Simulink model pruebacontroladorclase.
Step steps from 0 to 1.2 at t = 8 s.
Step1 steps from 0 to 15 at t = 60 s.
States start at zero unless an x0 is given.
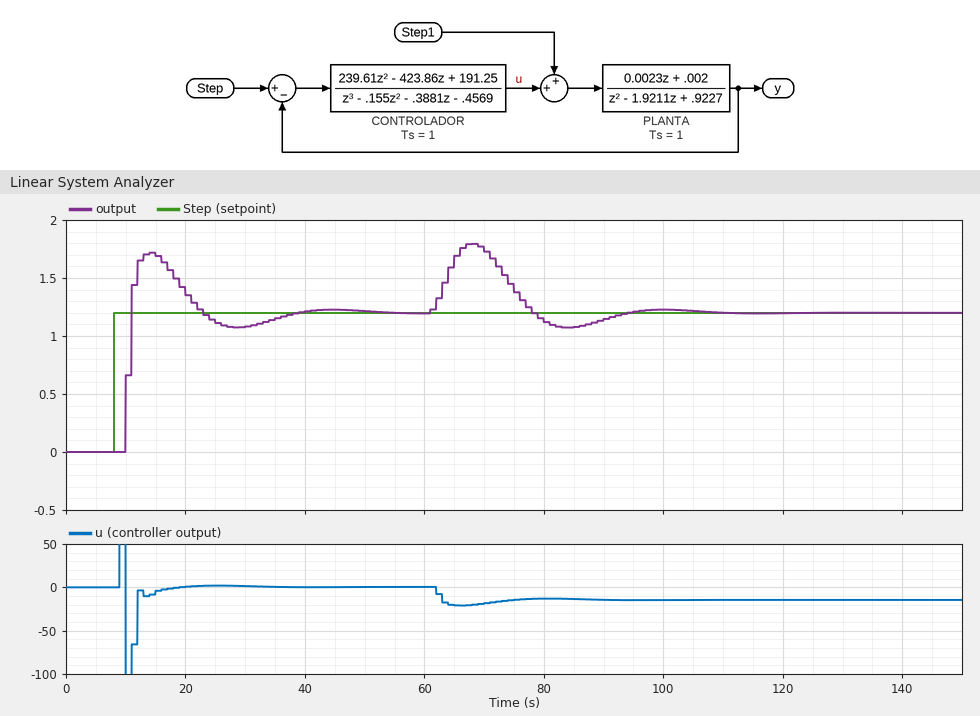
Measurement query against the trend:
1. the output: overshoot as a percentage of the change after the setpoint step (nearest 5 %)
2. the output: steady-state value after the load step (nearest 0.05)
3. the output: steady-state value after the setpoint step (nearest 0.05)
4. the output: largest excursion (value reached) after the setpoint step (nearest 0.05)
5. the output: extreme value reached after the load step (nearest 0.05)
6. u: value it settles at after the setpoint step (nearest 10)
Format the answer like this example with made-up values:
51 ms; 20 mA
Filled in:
45 %; 1.20; 1.20; 1.70; 1.80; 0
